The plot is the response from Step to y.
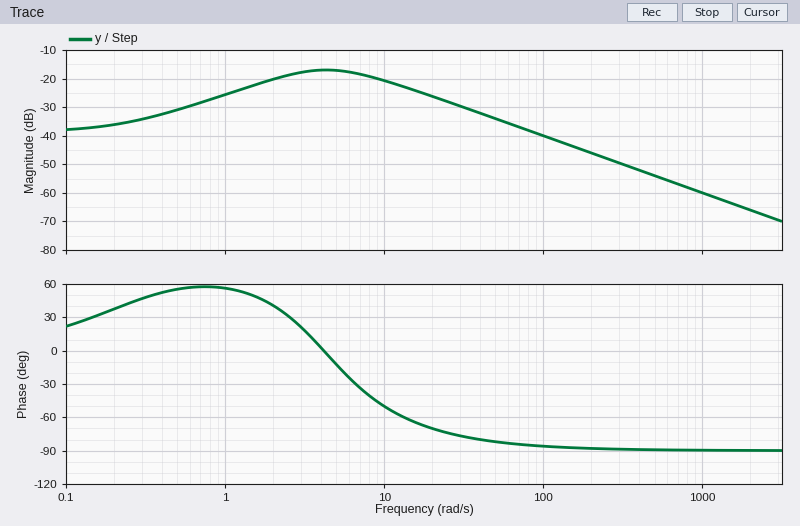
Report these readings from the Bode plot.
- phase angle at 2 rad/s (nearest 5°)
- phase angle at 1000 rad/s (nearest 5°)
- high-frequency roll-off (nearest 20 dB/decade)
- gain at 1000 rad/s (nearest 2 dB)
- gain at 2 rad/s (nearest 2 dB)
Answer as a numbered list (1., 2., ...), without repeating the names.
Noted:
1. 40°
2. -90°
3. -20 dB/decade
4. -60 dB
5. -20 dB
